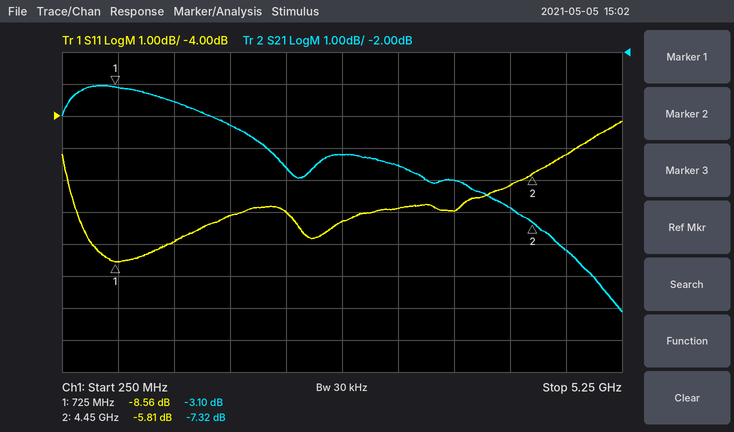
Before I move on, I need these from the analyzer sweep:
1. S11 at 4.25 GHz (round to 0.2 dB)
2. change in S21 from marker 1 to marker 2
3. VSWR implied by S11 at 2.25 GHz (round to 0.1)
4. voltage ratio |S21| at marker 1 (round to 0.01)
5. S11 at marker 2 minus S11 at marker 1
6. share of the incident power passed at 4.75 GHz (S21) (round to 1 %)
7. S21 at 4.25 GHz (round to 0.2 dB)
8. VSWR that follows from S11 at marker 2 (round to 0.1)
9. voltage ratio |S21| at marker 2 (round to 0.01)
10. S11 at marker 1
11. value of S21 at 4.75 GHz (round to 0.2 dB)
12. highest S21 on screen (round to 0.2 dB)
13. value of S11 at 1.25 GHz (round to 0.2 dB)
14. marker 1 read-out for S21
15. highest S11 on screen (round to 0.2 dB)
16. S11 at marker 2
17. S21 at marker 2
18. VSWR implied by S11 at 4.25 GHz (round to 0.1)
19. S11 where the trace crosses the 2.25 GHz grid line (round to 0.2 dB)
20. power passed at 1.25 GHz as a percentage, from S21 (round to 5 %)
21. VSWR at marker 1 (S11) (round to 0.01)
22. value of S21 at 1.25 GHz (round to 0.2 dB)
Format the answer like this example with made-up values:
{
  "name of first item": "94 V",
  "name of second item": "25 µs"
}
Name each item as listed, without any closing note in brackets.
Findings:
{
  "S11 at 4.25 GHz": "-6.2 dB",
  "change in S21 from marker 1 to marker 2": "-4.22 dB",
  "VSWR implied by S11 at 2.25 GHz": "2.6",
  "voltage ratio |S21| at marker 1": "0.70",
  "S11 at marker 2 minus S11 at marker 1": "2.75 dB",
  "share of the incident power passed at 4.75 GHz (S21)": "15 %",
  "S21 at 4.25 GHz": "-6.8 dB",
  "VSWR that follows from S11 at marker 2": "3.1",
  "voltage ratio |S21| at marker 2": "0.43",
  "S11 at marker 1": "-8.56 dB",
  "value of S21 at 4.75 GHz": "-8.2 dB",
  "highest S21 on screen": "-3.0 dB",
  "value of S11 at 1.25 GHz": "-8.0 dB",
  "marker 1 read-out for S21": "-3.10 dB",
  "highest S11 on screen": "-4.2 dB",
  "S11 at marker 2": "-5.81 dB",
  "S21 at marker 2": "-7.32 dB",
  "VSWR implied by S11 at 4.25 GHz": "2.9",
  "S11 where the trace crosses the 2.25 GHz grid line": "-7.0 dB",
  "power passed at 1.25 GHz as a percentage, from S21": "45 %",
  "VSWR at marker 1 (S11)": "2.19",
  "value of S21 at 1.25 GHz": "-3.6 dB"
}
